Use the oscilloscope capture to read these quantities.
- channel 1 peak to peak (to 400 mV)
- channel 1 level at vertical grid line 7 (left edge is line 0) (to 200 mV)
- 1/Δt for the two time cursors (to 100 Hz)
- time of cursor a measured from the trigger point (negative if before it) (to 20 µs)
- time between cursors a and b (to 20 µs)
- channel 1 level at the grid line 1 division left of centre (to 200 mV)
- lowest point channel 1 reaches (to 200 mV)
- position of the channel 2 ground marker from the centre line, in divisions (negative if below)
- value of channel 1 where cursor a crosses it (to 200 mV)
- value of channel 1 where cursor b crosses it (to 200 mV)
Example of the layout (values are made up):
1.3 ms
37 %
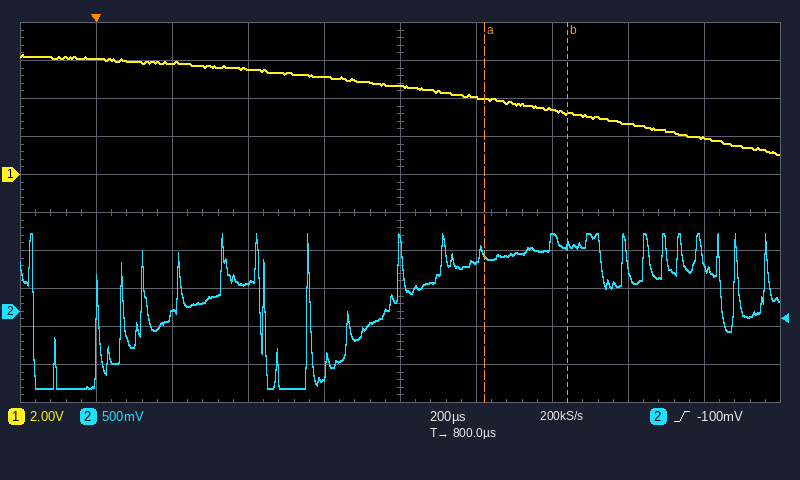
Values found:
5.2 V
3.4 V
4.5 kHz
+1.02 ms
220 µs
5.2 V
1.0 V
-2.6 div
4.0 V
3.2 V
